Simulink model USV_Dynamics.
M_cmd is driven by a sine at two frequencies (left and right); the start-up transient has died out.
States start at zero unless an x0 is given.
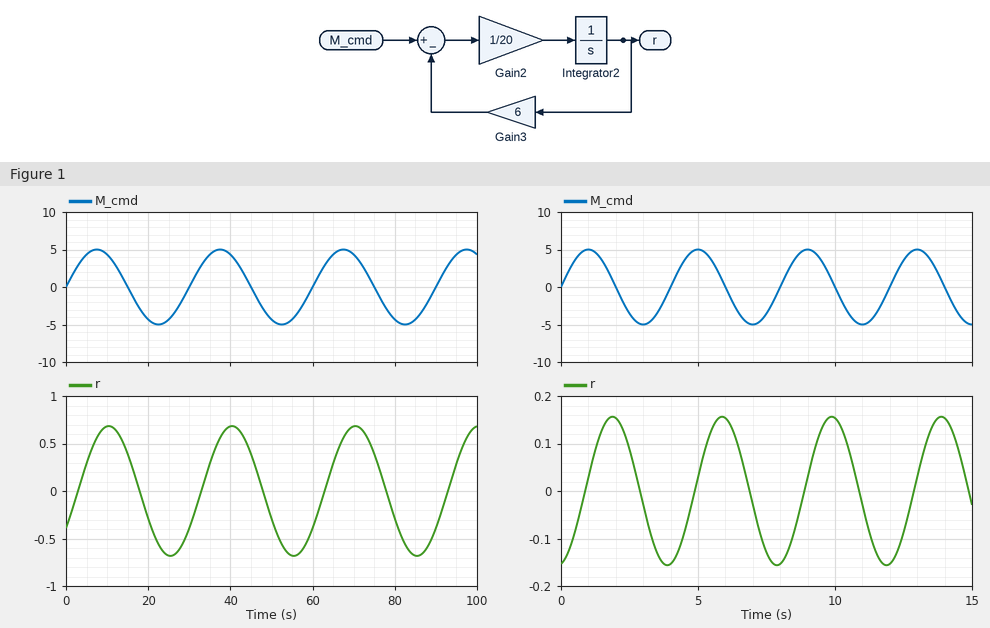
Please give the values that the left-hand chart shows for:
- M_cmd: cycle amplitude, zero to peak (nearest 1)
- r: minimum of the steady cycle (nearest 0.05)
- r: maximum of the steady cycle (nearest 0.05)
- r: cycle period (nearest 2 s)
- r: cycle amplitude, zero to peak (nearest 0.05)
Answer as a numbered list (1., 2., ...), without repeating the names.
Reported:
1. 5
2. -0.70
3. 0.70
4. 30 s
5. 0.70
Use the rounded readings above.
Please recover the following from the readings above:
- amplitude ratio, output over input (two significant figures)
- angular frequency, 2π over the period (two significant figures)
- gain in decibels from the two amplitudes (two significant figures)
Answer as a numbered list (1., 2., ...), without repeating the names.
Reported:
1. 0.14
2. 0.21 rad/s
3. -17 dB
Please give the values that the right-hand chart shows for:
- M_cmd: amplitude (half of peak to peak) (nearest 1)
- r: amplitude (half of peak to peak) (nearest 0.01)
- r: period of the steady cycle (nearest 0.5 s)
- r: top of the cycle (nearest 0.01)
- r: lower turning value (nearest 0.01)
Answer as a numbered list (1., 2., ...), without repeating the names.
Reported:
1. 5
2. 0.16
3. 4.0 s
4. 0.16
5. -0.16
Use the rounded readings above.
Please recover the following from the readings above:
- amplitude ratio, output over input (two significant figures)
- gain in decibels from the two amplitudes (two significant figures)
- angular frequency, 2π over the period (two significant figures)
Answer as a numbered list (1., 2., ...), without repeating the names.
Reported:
1. 0.032
2. -30 dB
3. 1.6 rad/s
